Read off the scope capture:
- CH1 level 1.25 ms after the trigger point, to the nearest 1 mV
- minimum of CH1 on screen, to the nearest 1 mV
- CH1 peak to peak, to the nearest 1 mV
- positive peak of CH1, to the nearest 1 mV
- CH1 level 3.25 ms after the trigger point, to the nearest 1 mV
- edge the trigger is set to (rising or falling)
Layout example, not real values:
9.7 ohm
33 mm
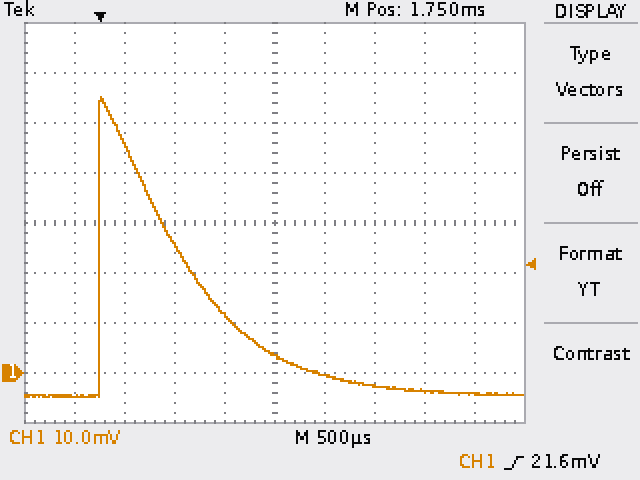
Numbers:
12 mV
-5 mV
60 mV
55 mV
-4 mV
rising
